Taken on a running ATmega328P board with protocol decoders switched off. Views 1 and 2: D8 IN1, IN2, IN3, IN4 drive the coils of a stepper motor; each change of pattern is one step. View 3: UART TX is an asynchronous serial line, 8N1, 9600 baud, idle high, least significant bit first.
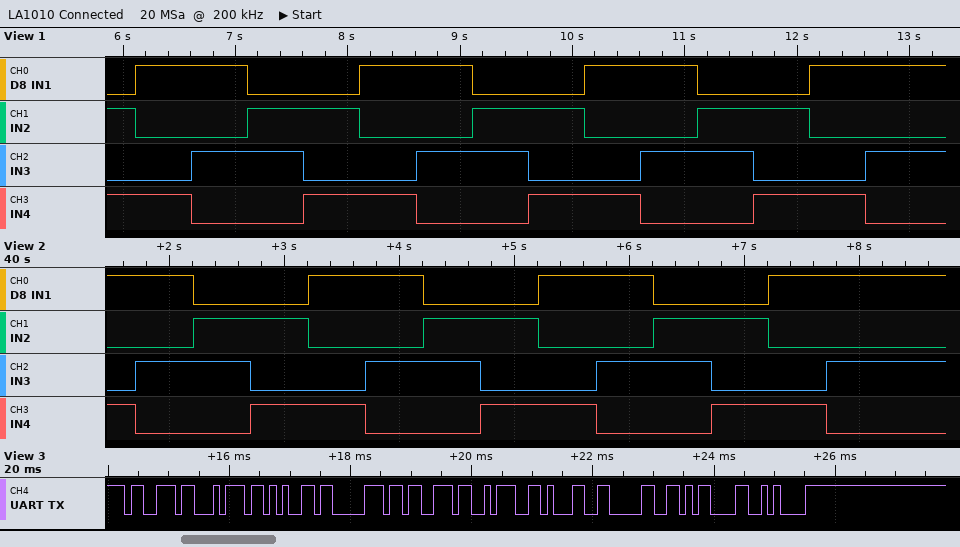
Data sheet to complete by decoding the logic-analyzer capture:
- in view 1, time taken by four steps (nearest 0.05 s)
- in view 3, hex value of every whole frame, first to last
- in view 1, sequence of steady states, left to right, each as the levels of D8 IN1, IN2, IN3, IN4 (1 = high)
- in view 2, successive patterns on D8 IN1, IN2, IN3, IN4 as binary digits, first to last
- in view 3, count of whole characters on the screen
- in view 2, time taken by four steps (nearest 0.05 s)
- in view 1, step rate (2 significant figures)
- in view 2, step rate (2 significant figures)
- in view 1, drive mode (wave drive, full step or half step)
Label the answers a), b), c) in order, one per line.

a) 2.00 s
b) 73 74 65 70 73 3A 31 30 0D 0A
c) 0101 1001 1010 0110 0101 1001 1010 0110 0101 1001 1010 0110 0101 1001 1010
d) 1001 1010 0110 0101 1001 1010 0110 0101 1001 1010 0110 0101 1001 1010
e) 10
f) 2.00 s
g) 2.0 steps/s
h) 2.0 steps/s
i) full step
